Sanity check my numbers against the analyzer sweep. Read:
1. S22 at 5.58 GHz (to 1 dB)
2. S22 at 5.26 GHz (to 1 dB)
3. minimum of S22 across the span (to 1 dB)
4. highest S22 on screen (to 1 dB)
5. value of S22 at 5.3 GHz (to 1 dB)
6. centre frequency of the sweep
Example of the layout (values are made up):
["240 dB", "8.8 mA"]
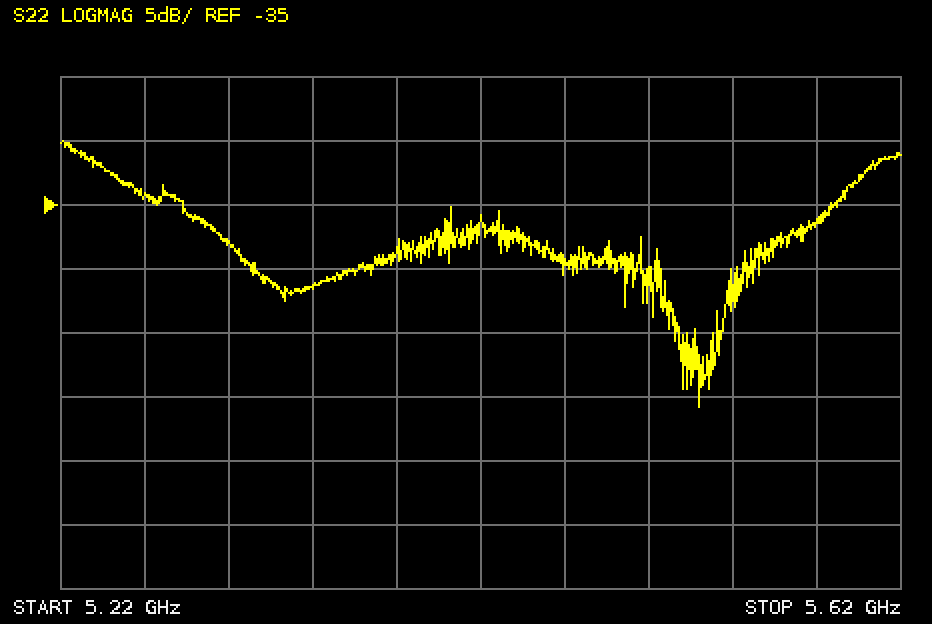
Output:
["-36 dB", "-34 dB", "-51 dB", "-30 dB", "-38 dB", "5.42 GHz"]
